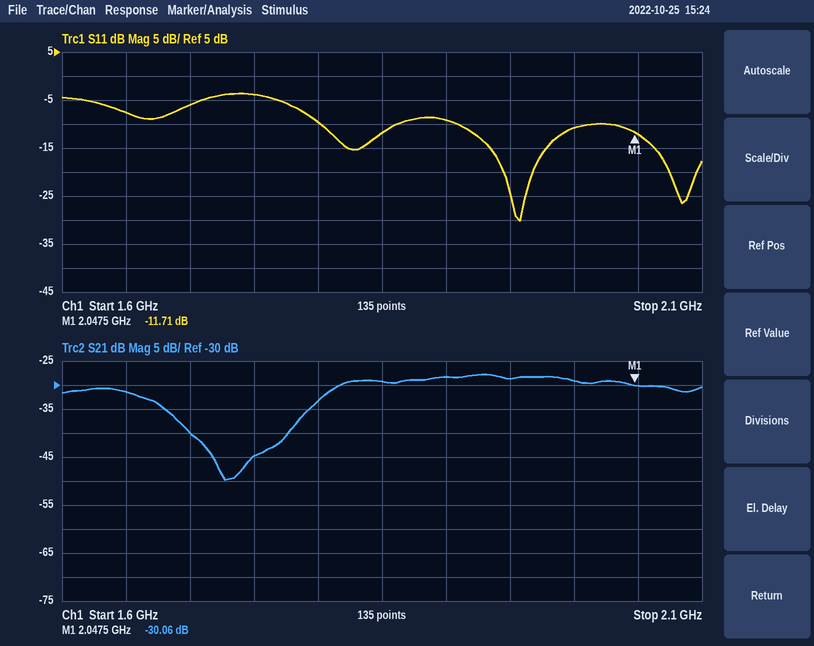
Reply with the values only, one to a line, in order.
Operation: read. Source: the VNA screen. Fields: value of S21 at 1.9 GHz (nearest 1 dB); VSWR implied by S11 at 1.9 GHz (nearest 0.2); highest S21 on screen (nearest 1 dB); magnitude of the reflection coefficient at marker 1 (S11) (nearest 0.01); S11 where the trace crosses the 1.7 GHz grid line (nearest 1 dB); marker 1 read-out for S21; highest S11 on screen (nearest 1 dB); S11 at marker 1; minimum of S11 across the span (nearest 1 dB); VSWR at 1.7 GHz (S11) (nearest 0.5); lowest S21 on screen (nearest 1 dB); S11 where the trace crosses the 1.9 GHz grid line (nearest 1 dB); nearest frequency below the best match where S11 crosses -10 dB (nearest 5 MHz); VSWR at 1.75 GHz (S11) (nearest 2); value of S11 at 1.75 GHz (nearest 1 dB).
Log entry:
-28 dB
2.0
-28 dB
0.26
-6 dB
-30.06 dB
-4 dB
-11.71 dB
-30 dB
3.0
-50 dB
-9 dB
1.910 GHz
4
-4 dB
